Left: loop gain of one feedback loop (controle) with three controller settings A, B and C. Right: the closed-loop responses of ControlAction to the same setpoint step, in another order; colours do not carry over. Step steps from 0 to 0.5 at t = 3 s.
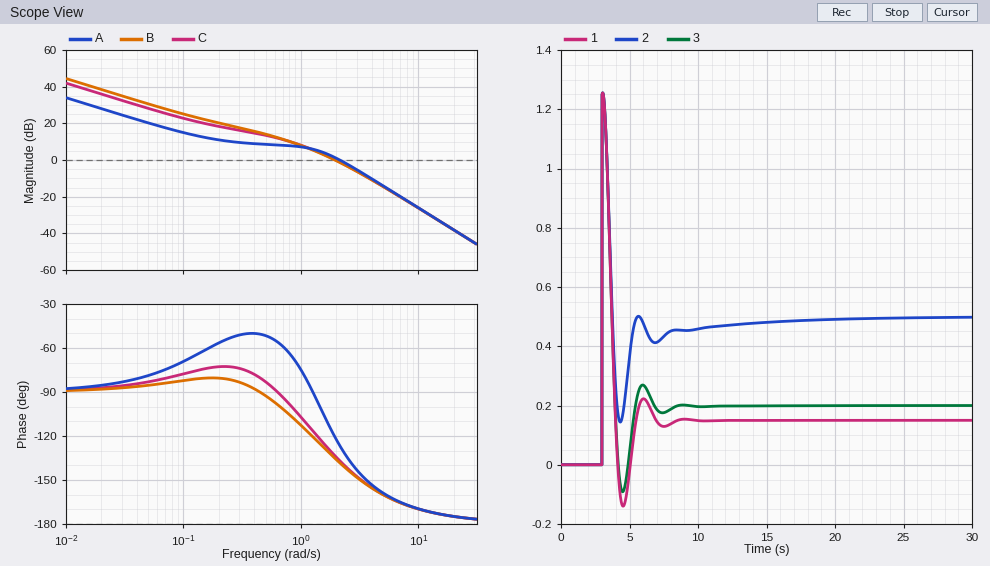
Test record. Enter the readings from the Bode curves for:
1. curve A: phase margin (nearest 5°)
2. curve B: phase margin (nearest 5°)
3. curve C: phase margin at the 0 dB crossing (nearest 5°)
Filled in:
55°
45°
45°
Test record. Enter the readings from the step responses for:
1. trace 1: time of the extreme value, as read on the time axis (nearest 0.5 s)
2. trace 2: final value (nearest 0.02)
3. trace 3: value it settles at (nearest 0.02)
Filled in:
3.0 s
0.50
0.20
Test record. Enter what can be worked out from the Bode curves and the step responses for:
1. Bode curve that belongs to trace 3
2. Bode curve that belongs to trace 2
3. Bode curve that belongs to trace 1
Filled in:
C
A
B
